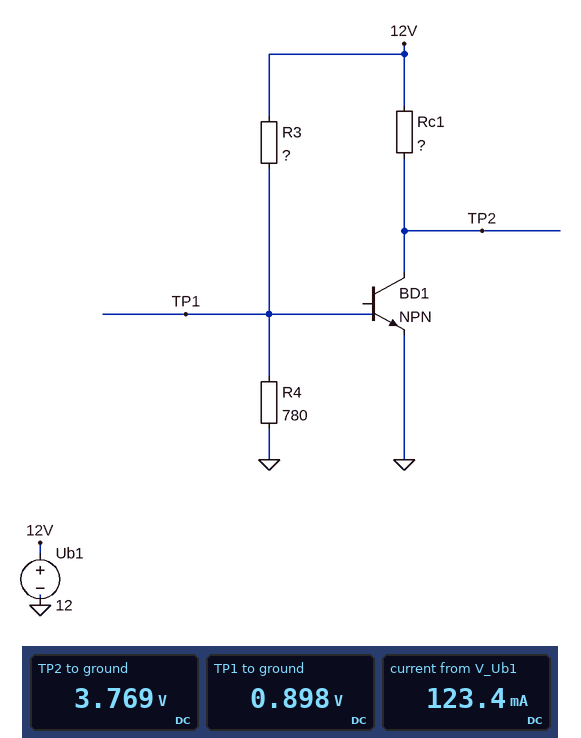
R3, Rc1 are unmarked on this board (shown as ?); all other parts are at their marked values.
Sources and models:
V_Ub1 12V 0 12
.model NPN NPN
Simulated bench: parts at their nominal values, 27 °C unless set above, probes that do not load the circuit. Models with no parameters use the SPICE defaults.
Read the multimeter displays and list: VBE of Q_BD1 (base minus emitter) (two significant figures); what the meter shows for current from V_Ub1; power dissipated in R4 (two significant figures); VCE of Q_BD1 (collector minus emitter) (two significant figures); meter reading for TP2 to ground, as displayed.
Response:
900 mV
123.4 mA
1.0 mW
3.8 V
3.769 V
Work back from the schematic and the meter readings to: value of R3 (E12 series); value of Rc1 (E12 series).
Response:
4.7 kΩ
68 Ω
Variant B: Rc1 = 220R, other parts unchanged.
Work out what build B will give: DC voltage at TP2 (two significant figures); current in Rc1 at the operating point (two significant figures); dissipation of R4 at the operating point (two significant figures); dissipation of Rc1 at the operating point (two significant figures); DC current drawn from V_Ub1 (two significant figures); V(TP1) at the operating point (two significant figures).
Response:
110 mV
54 mA
990 µW
640 mW
56 mA
880 mV
